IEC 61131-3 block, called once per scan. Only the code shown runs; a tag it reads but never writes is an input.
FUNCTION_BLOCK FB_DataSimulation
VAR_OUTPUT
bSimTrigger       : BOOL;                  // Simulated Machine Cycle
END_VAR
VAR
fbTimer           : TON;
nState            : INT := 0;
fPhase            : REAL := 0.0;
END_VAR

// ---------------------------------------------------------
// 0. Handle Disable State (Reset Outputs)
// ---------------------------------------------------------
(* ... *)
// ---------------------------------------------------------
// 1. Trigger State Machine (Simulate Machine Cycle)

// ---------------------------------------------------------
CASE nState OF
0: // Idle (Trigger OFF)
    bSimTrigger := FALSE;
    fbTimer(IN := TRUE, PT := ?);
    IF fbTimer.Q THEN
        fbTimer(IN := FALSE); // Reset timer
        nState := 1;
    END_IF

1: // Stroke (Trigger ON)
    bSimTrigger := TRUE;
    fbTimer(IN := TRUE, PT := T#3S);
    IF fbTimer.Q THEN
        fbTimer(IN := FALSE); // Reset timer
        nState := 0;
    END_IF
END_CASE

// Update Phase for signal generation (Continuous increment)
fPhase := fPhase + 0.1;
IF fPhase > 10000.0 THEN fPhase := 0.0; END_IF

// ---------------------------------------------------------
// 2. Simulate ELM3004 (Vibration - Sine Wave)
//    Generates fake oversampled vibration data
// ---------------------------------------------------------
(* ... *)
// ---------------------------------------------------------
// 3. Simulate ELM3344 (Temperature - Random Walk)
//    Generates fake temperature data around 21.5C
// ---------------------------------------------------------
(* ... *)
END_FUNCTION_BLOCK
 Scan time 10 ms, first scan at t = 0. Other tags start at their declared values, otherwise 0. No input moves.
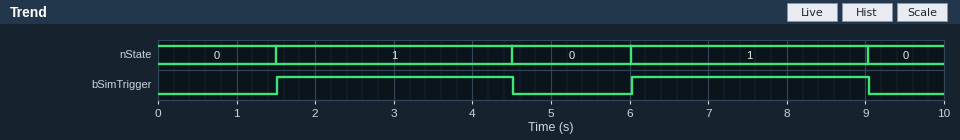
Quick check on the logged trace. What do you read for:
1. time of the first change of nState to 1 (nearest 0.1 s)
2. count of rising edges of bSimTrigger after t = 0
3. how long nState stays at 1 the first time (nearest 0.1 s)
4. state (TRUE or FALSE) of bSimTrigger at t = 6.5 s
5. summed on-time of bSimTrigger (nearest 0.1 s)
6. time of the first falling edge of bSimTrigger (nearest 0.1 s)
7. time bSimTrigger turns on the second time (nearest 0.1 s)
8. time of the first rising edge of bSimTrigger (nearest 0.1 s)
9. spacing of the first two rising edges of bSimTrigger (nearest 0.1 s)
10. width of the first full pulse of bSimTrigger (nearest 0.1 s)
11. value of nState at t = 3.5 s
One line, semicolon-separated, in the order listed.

1.5 s; 2; 3.0 s; TRUE; 6.0 s; 4.5 s; 6.0 s; 1.5 s; 4.5 s; 3.0 s; 1
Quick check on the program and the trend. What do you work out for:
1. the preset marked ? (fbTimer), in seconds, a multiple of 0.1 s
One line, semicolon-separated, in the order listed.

1.5 s
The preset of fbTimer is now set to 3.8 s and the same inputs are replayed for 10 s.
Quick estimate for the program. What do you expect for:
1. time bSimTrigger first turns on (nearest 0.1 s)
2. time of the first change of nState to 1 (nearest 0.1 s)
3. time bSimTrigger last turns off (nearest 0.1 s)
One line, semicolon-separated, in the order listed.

3.8 s; 3.8 s; 6.8 s
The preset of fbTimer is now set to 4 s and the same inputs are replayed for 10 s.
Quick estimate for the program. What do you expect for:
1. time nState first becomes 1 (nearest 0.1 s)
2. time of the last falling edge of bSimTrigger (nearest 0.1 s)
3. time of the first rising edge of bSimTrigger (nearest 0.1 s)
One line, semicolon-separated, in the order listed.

4.0 s; 7.0 s; 4.0 s
